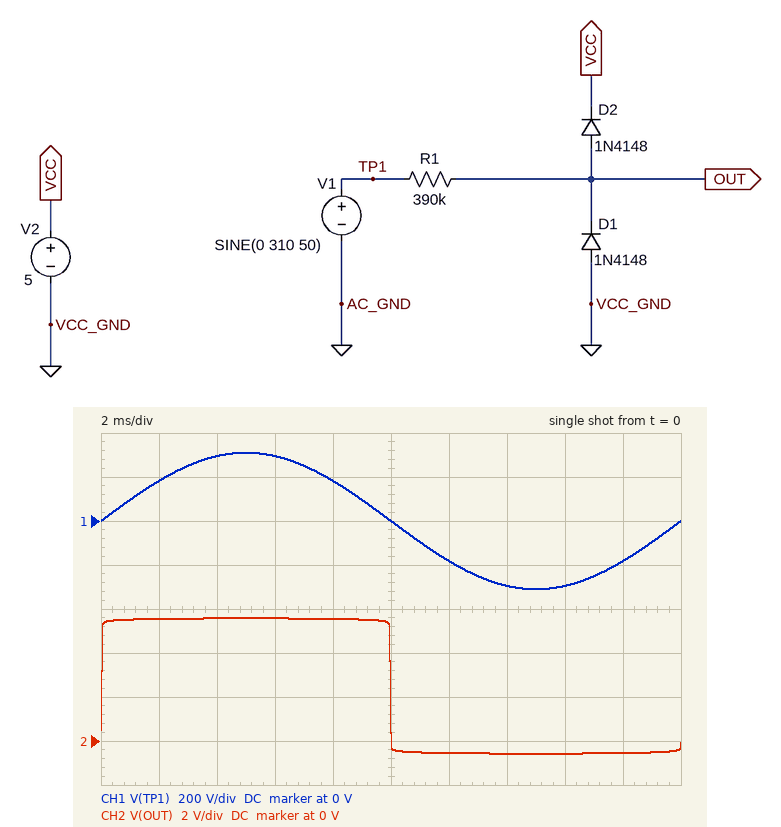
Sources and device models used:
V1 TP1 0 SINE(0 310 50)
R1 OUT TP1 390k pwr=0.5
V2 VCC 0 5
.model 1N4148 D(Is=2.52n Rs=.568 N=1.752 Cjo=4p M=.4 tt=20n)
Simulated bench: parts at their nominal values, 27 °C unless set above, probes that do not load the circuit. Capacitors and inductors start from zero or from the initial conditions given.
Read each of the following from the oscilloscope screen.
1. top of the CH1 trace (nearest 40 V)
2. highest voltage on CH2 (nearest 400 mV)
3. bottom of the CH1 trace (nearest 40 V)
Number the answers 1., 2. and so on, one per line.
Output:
1. 320 V
2. 5.6 V
3. -320 V
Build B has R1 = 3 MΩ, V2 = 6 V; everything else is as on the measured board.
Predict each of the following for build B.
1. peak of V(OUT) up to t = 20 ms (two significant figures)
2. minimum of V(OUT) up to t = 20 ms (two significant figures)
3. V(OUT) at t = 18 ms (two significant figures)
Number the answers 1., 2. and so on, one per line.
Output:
1. 6.5 V
2. -480 mV
3. -460 mV
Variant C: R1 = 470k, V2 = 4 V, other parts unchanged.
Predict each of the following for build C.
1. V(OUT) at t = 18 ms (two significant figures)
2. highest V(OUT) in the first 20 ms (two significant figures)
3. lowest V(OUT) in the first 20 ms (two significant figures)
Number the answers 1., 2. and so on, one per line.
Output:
1. -540 mV
2. 4.6 V
3. -570 mV
